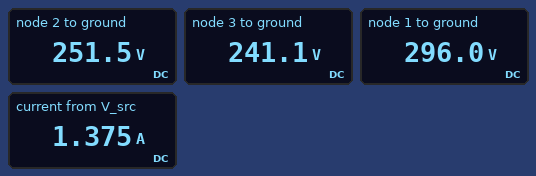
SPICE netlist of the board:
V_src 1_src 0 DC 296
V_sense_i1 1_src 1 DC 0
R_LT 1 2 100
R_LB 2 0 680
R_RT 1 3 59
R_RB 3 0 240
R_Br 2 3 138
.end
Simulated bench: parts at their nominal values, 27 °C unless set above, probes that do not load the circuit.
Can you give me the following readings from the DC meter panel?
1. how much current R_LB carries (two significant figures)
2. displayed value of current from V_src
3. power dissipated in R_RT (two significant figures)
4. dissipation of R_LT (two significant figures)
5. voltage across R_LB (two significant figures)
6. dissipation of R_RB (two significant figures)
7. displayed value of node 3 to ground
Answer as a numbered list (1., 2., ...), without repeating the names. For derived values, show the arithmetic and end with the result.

1. (251.5 V) / 680 Ω = 370 mA
2. 1.375 A
3. (296 V - 241.1 V)^2 / 59 Ω = 51 W
4. (296 V - 251.5 V)^2 / 100 Ω = 20 W
5. 251.5 V = 250 V
6. (241.1 V)^2 / 240 Ω = 240 W
7. 241.1 V
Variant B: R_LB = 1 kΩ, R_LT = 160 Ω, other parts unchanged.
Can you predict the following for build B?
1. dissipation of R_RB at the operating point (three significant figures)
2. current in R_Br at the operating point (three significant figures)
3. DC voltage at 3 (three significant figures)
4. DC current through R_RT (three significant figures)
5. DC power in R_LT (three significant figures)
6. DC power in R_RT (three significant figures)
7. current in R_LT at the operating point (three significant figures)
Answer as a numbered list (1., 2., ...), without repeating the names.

1. 240 W
2. 54.4 mA
3. 240 V
4. 946 mA
5. 14.6 W
6. 52.8 W
7. 302 mA
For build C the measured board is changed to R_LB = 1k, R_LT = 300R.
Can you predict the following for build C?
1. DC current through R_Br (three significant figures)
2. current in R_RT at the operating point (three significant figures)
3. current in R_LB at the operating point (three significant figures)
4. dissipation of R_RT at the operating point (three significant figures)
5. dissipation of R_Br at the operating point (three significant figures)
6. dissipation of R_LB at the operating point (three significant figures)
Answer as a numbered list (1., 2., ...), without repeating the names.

1. 23.8 mA
2. 1.01 A
3. 233 mA
4. 60.1 W
5. 78.1 mW
6. 54.4 W
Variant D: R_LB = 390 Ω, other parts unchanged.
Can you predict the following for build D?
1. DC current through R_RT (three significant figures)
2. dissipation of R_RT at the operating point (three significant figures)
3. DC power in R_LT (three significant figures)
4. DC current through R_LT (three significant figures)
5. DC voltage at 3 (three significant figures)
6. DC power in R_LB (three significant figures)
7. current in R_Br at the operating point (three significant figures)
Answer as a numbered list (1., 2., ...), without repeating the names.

1. 996 mA
2. 58.5 W
3. 35.8 W
4. 598 mA
5. 237 V
6. 143 W
7. 7.55 mA
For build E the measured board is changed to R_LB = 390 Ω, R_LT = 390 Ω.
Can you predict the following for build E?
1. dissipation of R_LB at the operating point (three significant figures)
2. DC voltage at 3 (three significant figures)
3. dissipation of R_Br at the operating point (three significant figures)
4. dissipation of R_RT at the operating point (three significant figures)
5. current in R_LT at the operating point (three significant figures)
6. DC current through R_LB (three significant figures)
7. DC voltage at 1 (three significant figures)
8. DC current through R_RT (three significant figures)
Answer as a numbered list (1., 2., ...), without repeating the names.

1. 96.4 W
2. 226 V
3. 7.66 W
4. 82.0 W
5. 262 mA
6. 497 mA
7. 296 V
8. 1.18 A
